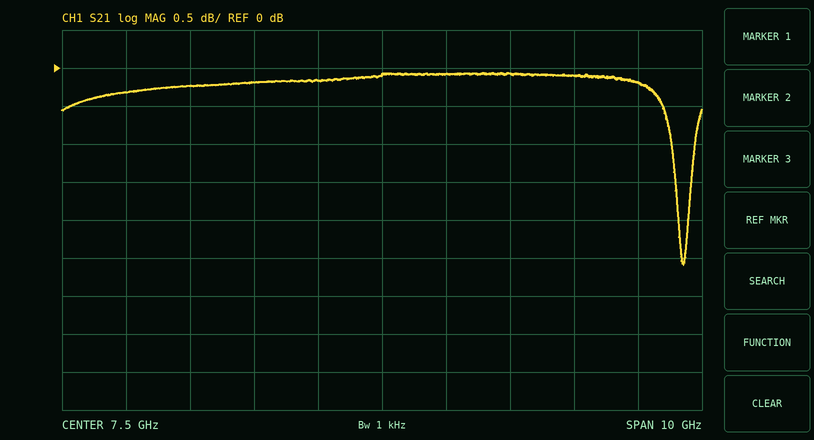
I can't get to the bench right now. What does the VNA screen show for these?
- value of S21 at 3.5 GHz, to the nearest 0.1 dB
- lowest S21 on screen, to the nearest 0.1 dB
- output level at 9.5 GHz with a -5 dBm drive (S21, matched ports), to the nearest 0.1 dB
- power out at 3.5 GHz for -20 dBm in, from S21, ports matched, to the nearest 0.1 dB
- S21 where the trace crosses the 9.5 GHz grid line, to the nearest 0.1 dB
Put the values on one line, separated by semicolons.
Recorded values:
-0.3 dB; -2.6 dB; -5.1 dBm; -20.3 dBm; -0.1 dB
